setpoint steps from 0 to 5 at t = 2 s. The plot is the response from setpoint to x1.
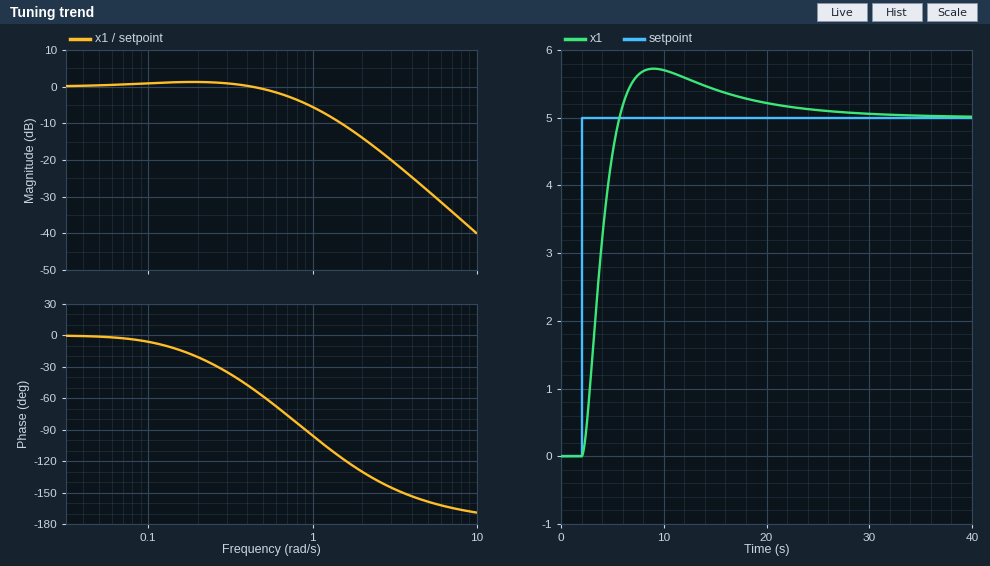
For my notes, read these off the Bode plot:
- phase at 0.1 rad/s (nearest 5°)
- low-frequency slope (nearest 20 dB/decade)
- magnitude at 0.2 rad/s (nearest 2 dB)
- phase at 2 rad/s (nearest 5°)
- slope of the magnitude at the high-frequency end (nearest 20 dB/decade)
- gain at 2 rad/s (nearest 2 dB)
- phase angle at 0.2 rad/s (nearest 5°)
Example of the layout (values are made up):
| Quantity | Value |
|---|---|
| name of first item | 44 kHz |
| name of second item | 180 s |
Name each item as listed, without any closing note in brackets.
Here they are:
| Quantity | Value |
|---|---|
| phase at 0.1 rad/s | -5° |
| low-frequency slope | 0 dB/decade |
| magnitude at 0.2 rad/s | 2 dB |
| phase at 2 rad/s | -130° |
| slope of the magnitude at the high-frequency end | -40 dB/decade |
| gain at 2 rad/s | -14 dB |
| phase angle at 0.2 rad/s | -20° |
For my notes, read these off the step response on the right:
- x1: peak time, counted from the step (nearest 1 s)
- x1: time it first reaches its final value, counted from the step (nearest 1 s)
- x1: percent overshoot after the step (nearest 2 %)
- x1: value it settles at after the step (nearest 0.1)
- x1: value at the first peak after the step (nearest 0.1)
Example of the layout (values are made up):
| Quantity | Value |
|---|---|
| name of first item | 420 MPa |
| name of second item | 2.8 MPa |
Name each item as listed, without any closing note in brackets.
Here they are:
| Quantity | Value |
|---|---|
| x1: peak time, counted from the step | 7 s |
| x1: time it first reaches its final value, counted from the step | 4 s |
| x1: percent overshoot after the step | 14 % |
| x1: value it settles at after the step | 5.0 |
| x1: value at the first peak after the step | 5.7 |
